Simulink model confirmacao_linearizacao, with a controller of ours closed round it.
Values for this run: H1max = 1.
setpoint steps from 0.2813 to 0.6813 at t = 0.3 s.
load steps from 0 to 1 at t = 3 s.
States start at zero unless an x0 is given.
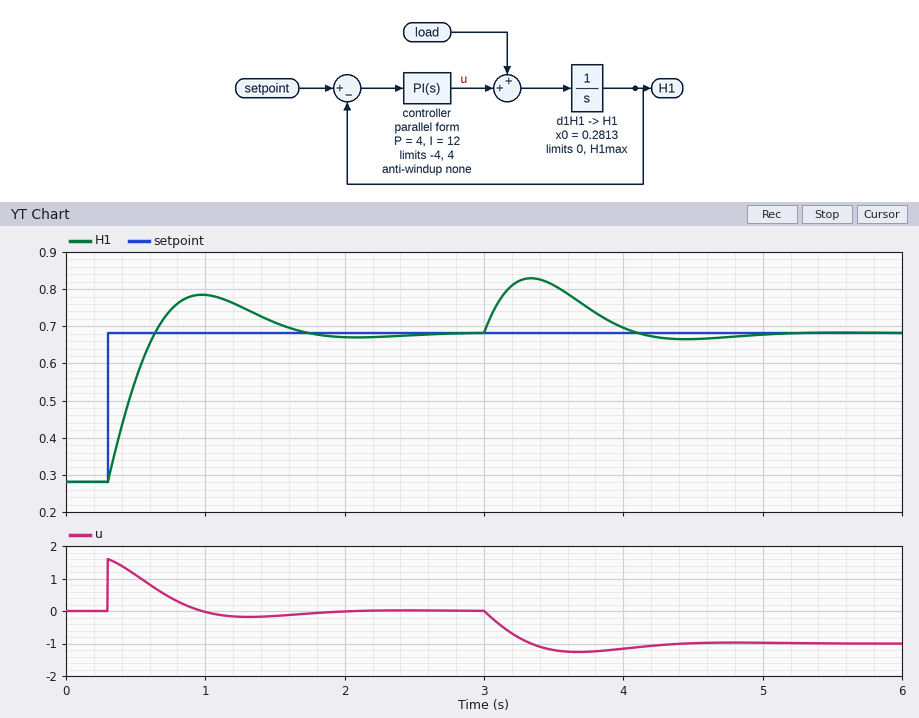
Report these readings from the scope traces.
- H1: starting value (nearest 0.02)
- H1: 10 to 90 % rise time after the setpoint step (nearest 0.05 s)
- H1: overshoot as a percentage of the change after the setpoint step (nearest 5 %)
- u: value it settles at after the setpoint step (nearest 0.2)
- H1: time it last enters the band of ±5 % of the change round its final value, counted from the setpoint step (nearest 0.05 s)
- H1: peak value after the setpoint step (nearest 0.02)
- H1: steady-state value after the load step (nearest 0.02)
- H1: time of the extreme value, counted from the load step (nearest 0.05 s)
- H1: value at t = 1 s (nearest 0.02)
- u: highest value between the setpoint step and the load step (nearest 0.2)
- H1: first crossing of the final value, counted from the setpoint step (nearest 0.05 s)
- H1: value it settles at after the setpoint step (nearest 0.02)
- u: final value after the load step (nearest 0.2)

0.28
0.25 s
25 %
0.0
1.25 s
0.78
0.68
0.35 s
0.78
1.6
0.35 s
0.68
-1.0
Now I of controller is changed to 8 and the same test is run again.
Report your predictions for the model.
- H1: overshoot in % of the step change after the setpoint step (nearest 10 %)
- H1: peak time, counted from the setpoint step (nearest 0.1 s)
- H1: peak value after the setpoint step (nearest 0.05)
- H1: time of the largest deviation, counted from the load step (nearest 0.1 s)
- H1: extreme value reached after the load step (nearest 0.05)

20 %
0.8 s
0.75
0.4 s
0.85
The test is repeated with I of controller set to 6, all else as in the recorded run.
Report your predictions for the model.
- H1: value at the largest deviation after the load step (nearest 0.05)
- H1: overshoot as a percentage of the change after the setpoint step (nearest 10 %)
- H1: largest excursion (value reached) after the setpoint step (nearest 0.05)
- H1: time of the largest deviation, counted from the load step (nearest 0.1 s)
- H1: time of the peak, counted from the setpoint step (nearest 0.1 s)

0.85
20 %
0.75
0.4 s
0.9 s
